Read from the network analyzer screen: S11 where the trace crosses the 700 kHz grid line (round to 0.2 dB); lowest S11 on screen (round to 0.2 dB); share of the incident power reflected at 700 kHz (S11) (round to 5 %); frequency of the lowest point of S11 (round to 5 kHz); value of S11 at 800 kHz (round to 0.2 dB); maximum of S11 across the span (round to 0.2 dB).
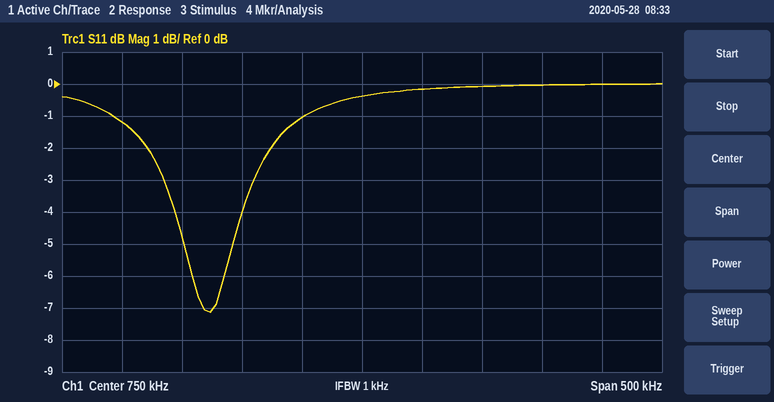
-1.0 dB
-7.2 dB
80 %
625 kHz
-0.2 dB
0.0 dB
